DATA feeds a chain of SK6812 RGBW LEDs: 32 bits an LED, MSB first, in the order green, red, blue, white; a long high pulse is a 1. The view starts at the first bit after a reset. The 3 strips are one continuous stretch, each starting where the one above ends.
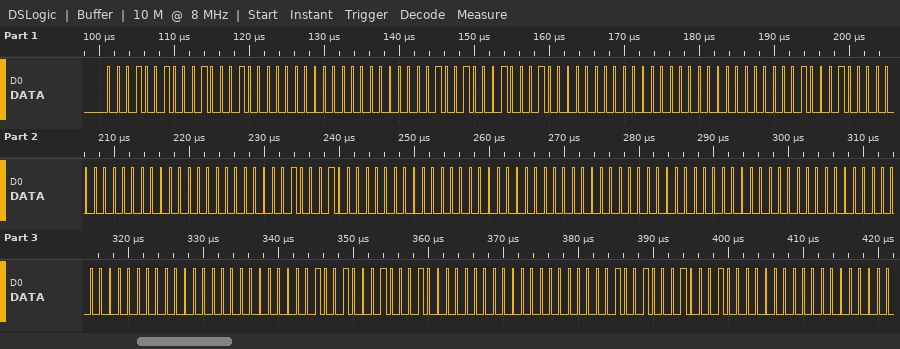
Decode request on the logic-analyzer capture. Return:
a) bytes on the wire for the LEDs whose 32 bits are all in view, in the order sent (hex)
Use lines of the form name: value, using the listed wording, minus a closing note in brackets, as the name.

bytes on the wire for the LEDs whose 32 bits are all in view, in the order sent: 12 22 00 00 12 22 00 00 00 22 00 00 00 22 00 00 00 00 00 00 00 00 00 00 12 22 00 00 12 22 00 00
